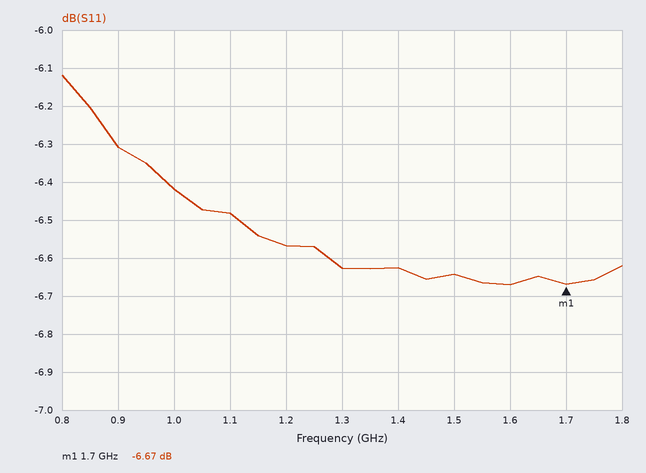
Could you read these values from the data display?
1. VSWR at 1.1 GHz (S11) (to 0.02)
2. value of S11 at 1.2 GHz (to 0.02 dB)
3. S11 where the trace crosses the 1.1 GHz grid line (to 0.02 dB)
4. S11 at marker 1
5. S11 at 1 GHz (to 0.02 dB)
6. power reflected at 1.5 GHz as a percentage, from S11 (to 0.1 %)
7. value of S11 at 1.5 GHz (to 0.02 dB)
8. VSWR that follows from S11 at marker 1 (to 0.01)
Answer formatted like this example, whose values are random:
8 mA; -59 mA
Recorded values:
2.80; -6.56 dB; -6.48 dB; -6.67 dB; -6.42 dB; 21.7 %; -6.64 dB; 2.73
